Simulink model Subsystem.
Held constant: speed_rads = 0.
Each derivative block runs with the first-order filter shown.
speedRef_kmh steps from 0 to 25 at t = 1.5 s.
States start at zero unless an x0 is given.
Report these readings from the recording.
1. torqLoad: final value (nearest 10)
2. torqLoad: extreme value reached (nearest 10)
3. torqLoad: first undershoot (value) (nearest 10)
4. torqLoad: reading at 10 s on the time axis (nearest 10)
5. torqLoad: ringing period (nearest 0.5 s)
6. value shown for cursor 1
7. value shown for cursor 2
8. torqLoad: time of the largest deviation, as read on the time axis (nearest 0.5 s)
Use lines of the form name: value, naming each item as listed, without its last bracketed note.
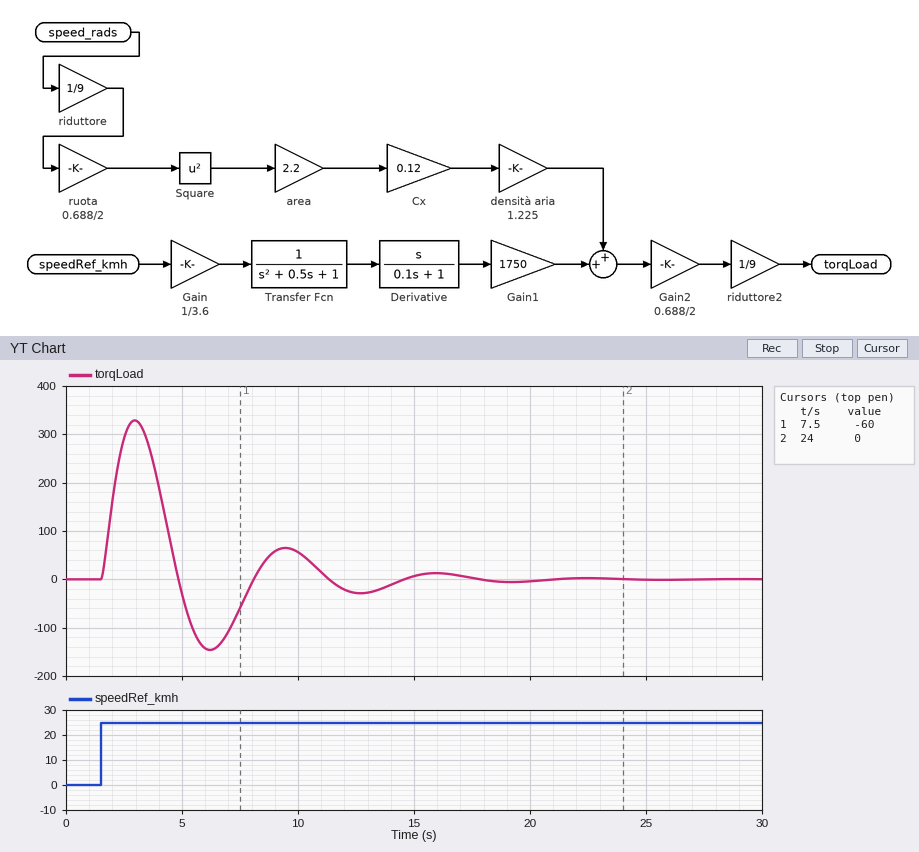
torqLoad: final value: 0
torqLoad: extreme value reached: 330
torqLoad: first undershoot (value): -150
torqLoad: reading at 10 s on the time axis: 60
torqLoad: ringing period: 6.5 s
value shown for cursor 1: -60
value shown for cursor 2: 0
torqLoad: time of the largest deviation, as read on the time axis: 3.0 s
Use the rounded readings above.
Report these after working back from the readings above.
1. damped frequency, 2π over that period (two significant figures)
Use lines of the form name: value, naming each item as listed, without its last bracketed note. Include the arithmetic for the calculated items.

damped frequency, 2π over that period: 2π / 6.5 = 0.97 rad/s
